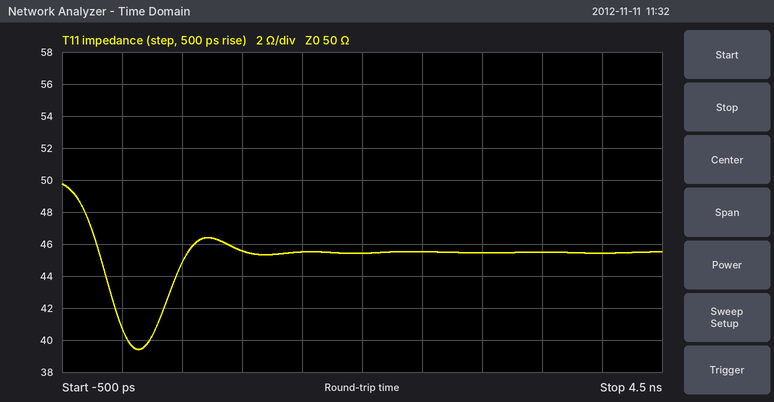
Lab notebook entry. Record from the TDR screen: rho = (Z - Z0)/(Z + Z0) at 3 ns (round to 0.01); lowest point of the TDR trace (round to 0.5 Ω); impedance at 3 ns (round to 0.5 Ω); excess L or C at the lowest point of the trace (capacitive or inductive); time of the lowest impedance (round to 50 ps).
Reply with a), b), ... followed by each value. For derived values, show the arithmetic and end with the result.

a) (45.5 − 50)/(45.5 + 50) ≈ -0.05
b) 39.5 Ω
c) 45.5 Ω
d) capacitive
e) 150 ps
